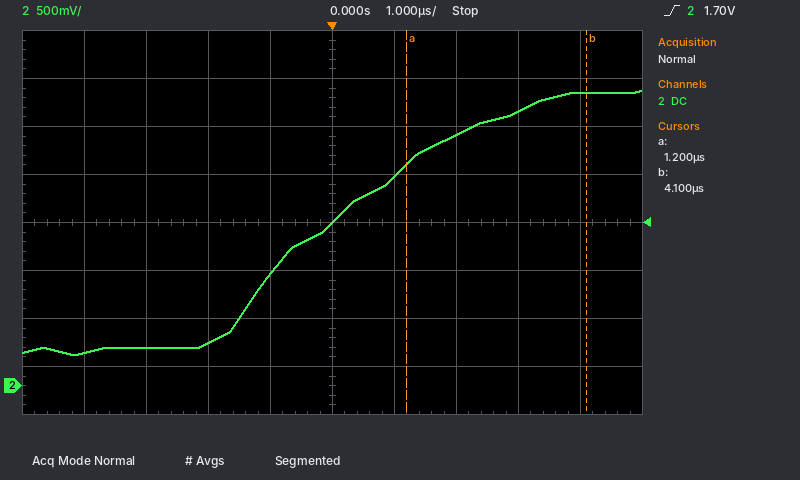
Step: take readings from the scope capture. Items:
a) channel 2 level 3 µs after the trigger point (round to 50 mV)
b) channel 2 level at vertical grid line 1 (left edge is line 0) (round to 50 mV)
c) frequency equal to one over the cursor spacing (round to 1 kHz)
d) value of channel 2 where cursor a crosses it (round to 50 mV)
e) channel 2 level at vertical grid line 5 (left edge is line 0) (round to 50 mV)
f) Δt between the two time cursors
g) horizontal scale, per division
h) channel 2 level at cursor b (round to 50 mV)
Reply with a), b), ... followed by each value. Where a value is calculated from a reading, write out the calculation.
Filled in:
a) 2.85 V
b) 350 mV
c) 1 / 2.9 µs ≈ 345 kHz
d) 2.30 V
e) 1.70 V
f) 4.1 µs − (1.2 µs) = 2.9 µs
g) 1 µs
h) 3.05 V
